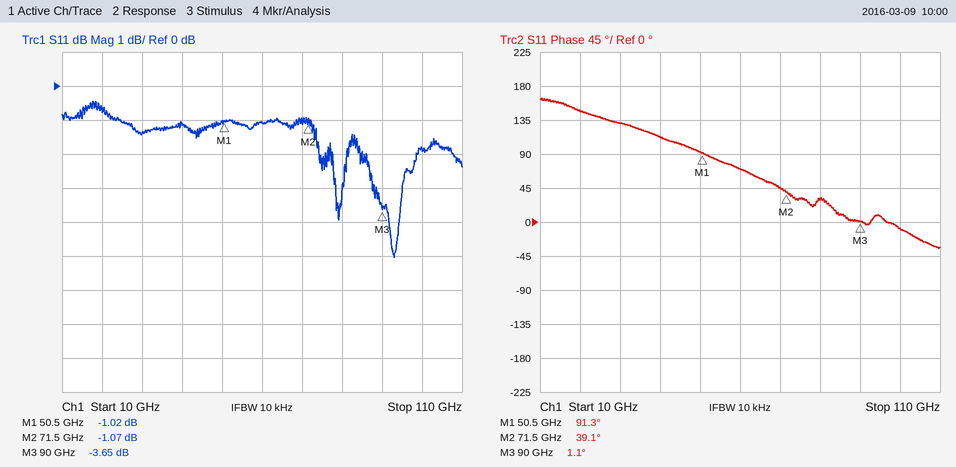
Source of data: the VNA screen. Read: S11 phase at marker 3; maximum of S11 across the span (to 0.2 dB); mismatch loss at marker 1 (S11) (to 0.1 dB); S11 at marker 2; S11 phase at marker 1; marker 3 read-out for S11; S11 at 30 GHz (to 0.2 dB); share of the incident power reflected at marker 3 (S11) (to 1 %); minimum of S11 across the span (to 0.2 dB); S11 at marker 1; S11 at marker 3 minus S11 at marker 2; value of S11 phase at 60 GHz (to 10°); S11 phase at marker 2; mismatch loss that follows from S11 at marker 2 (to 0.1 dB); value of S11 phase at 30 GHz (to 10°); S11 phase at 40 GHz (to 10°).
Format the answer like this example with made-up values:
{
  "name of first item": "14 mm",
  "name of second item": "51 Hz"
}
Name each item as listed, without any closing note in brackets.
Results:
{
  "S11 phase at marker 3": "1.1°",
  "maximum of S11 across the span": "-0.4 dB",
  "mismatch loss at marker 1 (S11)": "6.8 dB",
  "S11 at marker 2": "-1.07 dB",
  "S11 phase at marker 1": "91.3°",
  "marker 3 read-out for S11": "-3.65 dB",
  "S11 at 30 GHz": "-1.4 dB",
  "share of the incident power reflected at marker 3 (S11)": "43 %",
  "minimum of S11 across the span": "-5.0 dB",
  "S11 at marker 1": "-1.02 dB",
  "S11 at marker 3 minus S11 at marker 2": "-2.58 dB",
  "value of S11 phase at 60 GHz": "70°",
  "S11 phase at marker 2": "39.1°",
  "mismatch loss that follows from S11 at marker 2": "6.6 dB",
  "value of S11 phase at 30 GHz": "130°",
  "S11 phase at 40 GHz": "110°"
}
